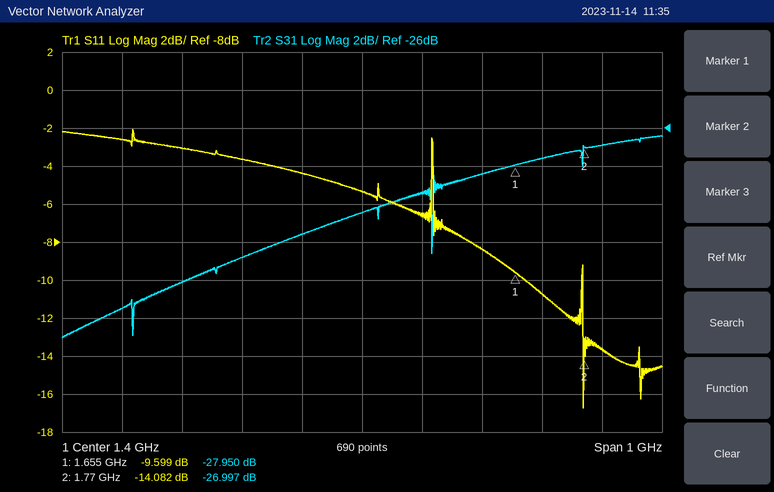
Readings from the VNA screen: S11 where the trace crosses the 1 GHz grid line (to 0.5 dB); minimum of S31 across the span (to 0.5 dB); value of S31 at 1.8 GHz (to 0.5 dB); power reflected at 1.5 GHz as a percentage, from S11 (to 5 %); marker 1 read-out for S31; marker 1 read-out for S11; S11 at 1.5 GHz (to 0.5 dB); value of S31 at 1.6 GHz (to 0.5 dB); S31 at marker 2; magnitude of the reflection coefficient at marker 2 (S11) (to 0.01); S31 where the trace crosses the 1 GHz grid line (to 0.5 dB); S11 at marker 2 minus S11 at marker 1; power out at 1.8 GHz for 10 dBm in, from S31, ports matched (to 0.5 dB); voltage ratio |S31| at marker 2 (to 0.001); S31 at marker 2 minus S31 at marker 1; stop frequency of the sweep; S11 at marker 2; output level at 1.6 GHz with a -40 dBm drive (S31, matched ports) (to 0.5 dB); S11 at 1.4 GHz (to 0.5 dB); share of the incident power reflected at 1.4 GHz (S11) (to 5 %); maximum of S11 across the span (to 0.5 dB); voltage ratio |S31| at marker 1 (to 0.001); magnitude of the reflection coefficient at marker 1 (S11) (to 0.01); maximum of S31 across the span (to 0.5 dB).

-2.5 dB
-37.0 dB
-27.0 dB
20 %
-27.950 dB
-9.599 dB
-6.5 dB
-28.5 dB
-26.997 dB
0.20
-35.5 dB
-4.483 dB
-17.0 dBm
0.045
0.953 dB
1.9 GHz
-14.082 dB
-68.5 dBm
-5.5 dB
30 %
-2.0 dB
0.040
0.33
-26.5 dB
